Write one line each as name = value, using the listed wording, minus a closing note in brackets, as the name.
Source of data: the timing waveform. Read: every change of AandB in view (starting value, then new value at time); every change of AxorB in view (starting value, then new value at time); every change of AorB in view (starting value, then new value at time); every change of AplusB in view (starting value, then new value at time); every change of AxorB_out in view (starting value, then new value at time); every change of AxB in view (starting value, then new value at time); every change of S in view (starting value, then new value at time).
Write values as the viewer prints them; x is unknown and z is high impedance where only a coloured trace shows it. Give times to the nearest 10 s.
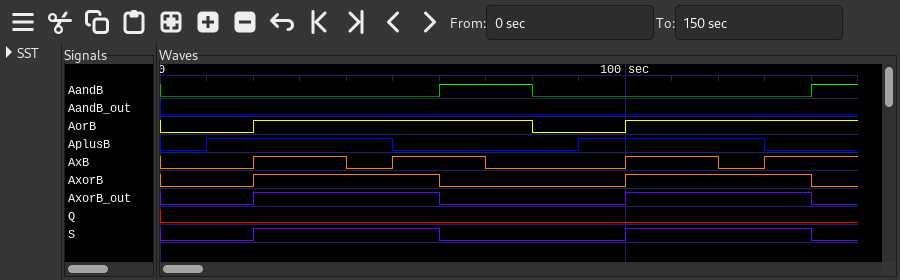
every change of AandB in view = 0, 1 at 60 s, 0 at 80 s, 1 at 140 s
every change of AxorB in view = 0, 1 at 20 s, 0 at 60 s, 1 at 100 s, 0 at 140 s
every change of AorB in view = 0, 1 at 20 s, 0 at 80 s, 1 at 100 s
every change of AplusB in view = 0, 1 at 10 s, 0 at 50 s, 1 at 90 s, 0 at 130 s
every change of AxorB_out in view = 0, 1 at 20 s, 0 at 60 s, 1 at 100 s, 0 at 140 s
every change of AxB in view = 0, 1 at 20 s, 0 at 40 s, 1 at 50 s, 0 at 70 s, 1 at 100 s, 0 at 120 s, 1 at 130 s
every change of S in view = 0, 1 at 20 s, 0 at 60 s, 1 at 100 s, 0 at 140 s
